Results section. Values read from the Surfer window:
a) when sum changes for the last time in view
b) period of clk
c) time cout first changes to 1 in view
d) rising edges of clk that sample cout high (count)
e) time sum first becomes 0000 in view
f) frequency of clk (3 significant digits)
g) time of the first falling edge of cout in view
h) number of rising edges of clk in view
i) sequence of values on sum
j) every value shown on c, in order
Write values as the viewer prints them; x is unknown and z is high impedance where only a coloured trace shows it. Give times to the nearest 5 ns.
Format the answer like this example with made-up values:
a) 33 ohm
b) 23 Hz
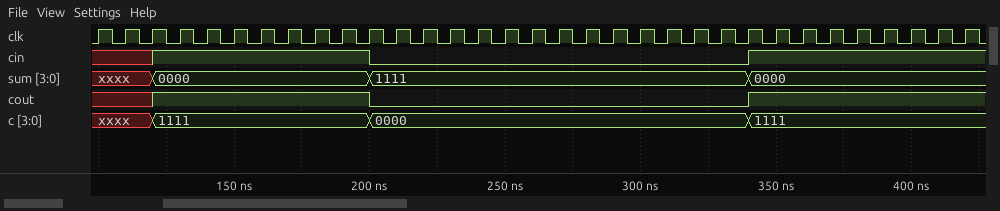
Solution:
a) 340 ns
b) 10 ns
c) 120 ns
d) 16
e) 120 ns
f) 100 MHz
g) 200 ns
h) 33
i) xxxx, 0000, 1111, 0000
j) xxxx, 1111, 0000, 1111
